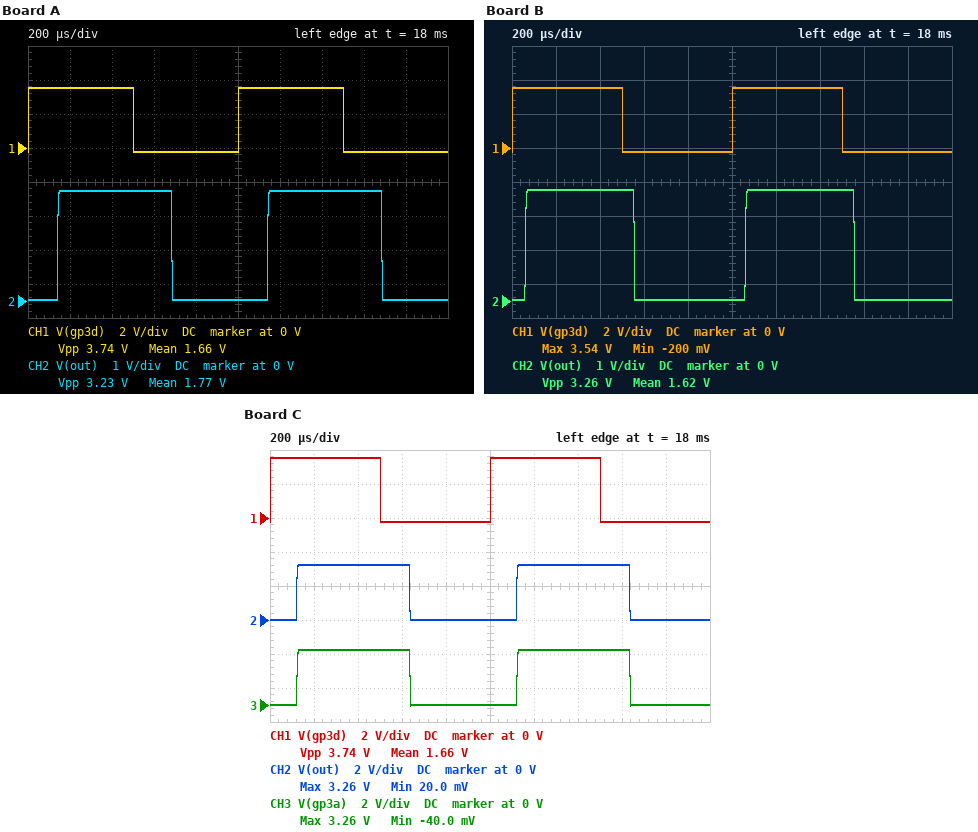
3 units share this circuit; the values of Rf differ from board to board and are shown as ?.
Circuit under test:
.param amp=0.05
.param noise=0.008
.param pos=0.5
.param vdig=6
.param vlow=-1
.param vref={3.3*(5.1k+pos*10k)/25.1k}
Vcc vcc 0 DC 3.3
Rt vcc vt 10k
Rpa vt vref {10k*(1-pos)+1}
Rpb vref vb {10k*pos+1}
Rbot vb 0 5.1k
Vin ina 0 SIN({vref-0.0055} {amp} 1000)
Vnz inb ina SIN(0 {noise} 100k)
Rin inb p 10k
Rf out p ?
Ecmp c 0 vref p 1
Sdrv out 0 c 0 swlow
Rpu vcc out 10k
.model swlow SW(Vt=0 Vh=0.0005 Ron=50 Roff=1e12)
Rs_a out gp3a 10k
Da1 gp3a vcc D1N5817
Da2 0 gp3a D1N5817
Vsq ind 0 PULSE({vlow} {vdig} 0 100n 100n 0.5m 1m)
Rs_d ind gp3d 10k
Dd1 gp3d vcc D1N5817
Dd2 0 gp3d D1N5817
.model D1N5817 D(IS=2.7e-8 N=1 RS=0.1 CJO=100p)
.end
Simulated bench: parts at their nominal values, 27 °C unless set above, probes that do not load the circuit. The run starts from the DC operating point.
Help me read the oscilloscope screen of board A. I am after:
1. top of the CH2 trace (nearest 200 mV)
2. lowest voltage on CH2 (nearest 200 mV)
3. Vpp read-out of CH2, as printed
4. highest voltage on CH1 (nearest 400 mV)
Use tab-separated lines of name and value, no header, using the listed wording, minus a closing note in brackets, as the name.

top of the CH2 trace	3.2 V
lowest voltage on CH2	0 V
Vpp read-out of CH2, as printed	3.23 V
highest voltage on CH1	3.6 V
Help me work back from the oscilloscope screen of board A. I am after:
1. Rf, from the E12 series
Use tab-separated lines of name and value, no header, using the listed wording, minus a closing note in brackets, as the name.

Rf, from the E12 series	330 kΩ
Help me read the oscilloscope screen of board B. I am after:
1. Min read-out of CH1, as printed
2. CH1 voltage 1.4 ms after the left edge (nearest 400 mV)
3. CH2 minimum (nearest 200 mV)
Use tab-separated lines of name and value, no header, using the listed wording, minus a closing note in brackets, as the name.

Min read-out of CH1, as printed	-200 mV
CH1 voltage 1.4 ms after the left edge	3.6 V
CH2 minimum	0 V
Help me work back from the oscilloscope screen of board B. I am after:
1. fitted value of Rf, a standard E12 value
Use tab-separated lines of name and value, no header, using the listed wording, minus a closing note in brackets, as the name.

fitted value of Rf, a standard E12 value	680 kΩ
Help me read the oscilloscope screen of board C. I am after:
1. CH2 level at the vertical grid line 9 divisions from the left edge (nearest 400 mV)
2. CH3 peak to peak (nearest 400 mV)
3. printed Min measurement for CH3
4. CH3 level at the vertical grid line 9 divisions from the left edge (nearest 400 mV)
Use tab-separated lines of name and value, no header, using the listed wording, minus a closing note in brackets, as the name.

CH2 level at the vertical grid line 9 divisions from the left edge	0 V
CH3 peak to peak	3.2 V
printed Min measurement for CH3	-40.0 mV
CH3 level at the vertical grid line 9 divisions from the left edge	0 V
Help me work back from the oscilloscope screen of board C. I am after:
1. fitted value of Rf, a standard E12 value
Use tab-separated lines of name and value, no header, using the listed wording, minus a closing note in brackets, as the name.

fitted value of Rf, a standard E12 value	390 kΩ
